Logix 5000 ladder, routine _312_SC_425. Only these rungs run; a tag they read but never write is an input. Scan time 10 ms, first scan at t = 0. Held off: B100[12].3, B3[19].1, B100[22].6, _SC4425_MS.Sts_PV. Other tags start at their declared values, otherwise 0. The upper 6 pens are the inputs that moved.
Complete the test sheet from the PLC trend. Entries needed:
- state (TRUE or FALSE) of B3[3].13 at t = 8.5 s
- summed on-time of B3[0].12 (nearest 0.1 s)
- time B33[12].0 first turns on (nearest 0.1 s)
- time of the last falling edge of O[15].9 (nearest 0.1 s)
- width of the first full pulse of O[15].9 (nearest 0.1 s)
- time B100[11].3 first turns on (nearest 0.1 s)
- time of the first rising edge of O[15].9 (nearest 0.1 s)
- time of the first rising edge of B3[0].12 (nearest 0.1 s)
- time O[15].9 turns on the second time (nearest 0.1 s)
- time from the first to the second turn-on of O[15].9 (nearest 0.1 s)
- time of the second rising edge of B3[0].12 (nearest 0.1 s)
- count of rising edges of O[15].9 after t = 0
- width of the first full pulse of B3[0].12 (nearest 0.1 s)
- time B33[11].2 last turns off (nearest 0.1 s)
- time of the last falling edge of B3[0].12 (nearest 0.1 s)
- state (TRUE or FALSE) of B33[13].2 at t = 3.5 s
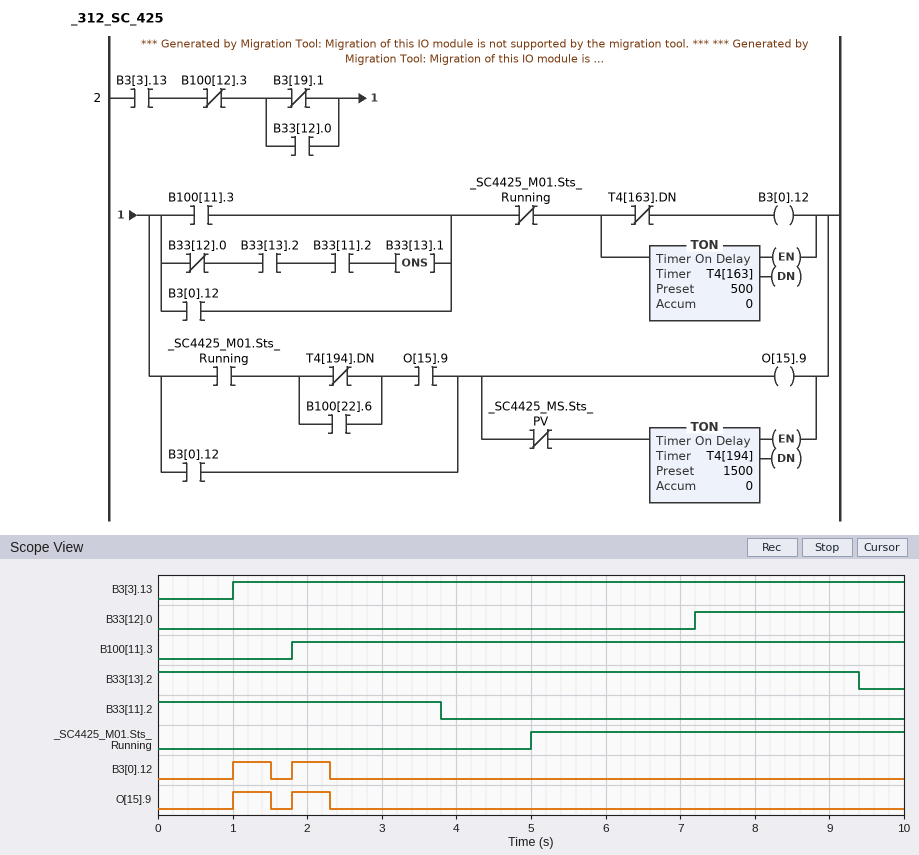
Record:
TRUE
1.0 s
7.2 s
2.3 s
0.5 s
1.8 s
1.0 s
1.0 s
1.8 s
0.8 s
1.8 s
2
0.5 s
3.8 s
2.3 s
TRUE
